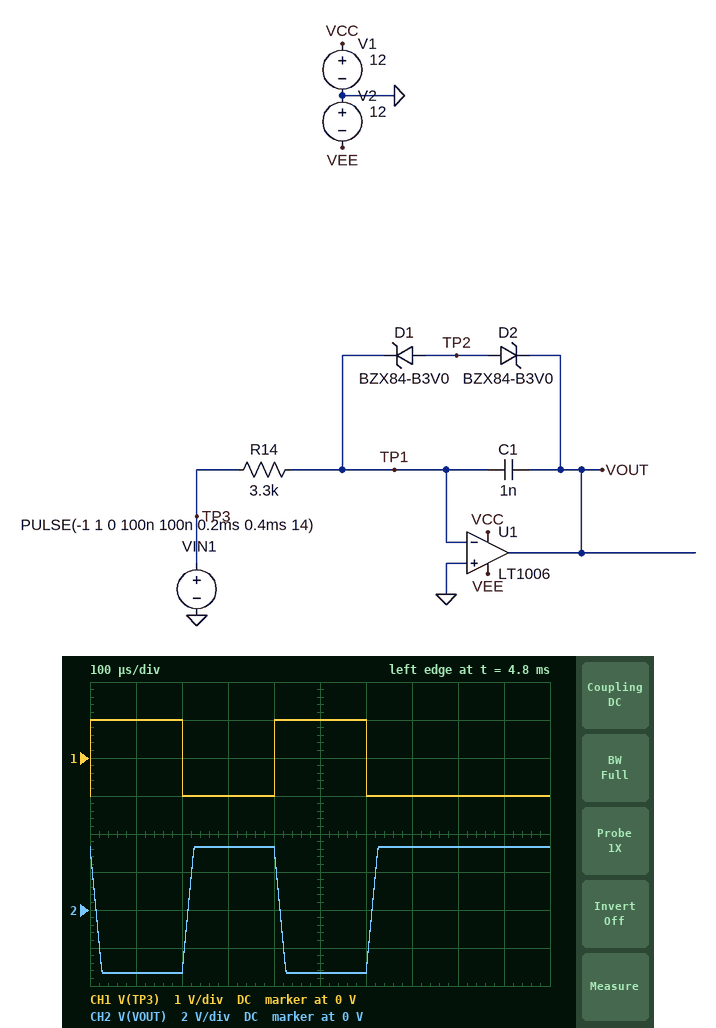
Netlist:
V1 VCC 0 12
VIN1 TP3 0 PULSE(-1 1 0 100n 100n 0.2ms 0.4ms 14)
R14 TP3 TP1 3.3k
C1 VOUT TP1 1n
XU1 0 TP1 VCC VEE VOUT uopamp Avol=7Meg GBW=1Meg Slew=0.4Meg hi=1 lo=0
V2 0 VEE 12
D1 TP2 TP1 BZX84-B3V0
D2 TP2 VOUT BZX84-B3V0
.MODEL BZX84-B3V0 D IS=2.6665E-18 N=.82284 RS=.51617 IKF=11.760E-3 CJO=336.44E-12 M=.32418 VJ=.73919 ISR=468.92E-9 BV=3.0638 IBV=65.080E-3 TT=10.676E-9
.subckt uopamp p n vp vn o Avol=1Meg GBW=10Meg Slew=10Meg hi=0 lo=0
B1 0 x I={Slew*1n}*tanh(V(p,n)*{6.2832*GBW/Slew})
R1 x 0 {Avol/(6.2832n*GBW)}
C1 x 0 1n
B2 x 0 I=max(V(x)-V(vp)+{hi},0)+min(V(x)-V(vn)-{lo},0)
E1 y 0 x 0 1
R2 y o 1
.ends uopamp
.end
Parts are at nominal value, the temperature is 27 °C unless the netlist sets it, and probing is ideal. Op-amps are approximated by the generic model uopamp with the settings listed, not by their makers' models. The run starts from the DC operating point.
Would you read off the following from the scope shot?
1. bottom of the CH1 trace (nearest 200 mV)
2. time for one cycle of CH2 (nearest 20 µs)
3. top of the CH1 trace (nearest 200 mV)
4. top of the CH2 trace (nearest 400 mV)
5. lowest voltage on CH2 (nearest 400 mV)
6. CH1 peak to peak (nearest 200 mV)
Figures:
-1.0 V
400 µs
1.0 V
3.2 V
-3.2 V
2.0 V
